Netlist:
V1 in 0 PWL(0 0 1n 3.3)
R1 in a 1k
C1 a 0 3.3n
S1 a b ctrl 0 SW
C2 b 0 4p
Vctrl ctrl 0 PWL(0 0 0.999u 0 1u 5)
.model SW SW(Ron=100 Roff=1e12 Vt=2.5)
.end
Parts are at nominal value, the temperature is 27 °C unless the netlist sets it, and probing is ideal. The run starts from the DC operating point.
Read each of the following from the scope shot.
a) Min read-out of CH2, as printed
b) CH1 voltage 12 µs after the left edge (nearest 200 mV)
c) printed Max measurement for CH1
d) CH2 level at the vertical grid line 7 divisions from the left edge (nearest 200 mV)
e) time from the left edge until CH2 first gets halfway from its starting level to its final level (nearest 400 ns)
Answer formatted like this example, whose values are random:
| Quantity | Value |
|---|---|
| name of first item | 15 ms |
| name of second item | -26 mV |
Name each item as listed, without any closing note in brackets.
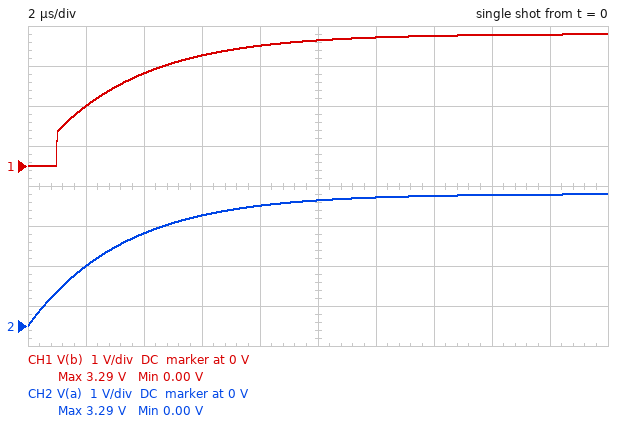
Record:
| Quantity | Value |
|---|---|
| Min read-out of CH2, as printed | 0.00 V |
| CH1 voltage 12 µs after the left edge | 3.2 V |
| printed Max measurement for CH1 | 3.29 V |
| CH2 level at the vertical grid line 7 divisions from the left edge | 3.2 V |
| time from the left edge until CH2 first gets halfway from its starting level to its final level | 2.4 µs |
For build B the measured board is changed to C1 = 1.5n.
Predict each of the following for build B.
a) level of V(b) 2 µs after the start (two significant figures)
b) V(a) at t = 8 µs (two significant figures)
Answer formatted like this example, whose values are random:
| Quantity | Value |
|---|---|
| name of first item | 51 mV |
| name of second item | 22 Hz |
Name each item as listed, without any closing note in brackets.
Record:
| Quantity | Value |
|---|---|
| level of V(b) 2 µs after the start | 2.4 V |
| V(a) at t = 8 µs | 3.3 V |
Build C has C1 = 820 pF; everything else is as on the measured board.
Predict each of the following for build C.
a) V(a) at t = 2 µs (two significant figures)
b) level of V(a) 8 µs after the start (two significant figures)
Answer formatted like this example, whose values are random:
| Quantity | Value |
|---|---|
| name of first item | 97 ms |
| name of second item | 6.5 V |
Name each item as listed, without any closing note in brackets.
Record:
| Quantity | Value |
|---|---|
| V(a) at t = 2 µs | 3.0 V |
| level of V(a) 8 µs after the start | 3.3 V |
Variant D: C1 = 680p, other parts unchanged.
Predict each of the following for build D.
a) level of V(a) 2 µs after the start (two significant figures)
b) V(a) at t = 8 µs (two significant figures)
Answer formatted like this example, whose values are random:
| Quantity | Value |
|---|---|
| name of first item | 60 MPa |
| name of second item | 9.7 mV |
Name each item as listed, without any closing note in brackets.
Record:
| Quantity | Value |
|---|---|
| level of V(a) 2 µs after the start | 3.1 V |
| V(a) at t = 8 µs | 3.3 V |
